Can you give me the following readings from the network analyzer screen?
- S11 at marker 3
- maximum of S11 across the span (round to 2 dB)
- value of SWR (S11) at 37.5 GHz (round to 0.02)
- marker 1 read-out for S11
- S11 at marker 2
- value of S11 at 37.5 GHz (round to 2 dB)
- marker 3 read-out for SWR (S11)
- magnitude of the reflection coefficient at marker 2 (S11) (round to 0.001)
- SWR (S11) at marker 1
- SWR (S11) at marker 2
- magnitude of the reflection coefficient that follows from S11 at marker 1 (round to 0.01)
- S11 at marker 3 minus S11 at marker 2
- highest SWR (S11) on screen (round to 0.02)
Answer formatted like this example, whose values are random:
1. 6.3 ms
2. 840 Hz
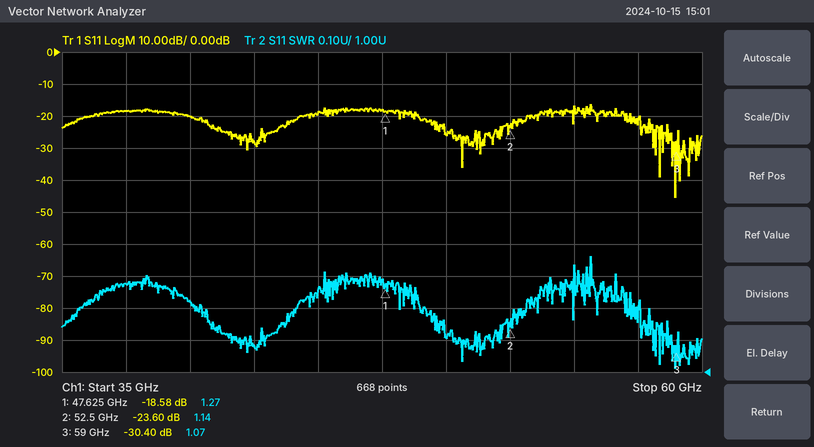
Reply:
1. -30.40 dB
2. -16 dB
3. 1.28
4. -18.58 dB
5. -23.60 dB
6. -18 dB
7. 1.07
8. 0.066
9. 1.27
10. 1.14
11. 0.12
12. -6.80 dB
13. 1.36
